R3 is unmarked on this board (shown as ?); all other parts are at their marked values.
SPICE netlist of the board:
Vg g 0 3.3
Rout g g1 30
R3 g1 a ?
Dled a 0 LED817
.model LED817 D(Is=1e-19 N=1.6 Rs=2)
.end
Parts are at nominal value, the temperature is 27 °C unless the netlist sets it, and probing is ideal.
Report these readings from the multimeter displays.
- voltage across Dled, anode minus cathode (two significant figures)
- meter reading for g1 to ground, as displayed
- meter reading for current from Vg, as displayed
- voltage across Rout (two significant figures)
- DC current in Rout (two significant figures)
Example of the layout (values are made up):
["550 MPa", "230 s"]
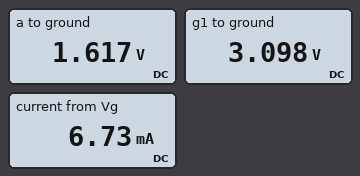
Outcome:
["1.6 V", "3.098 V", "6.73 mA", "200 mV", "6.7 mA"]
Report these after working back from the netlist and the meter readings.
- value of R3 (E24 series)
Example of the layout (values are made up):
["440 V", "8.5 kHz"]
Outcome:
["220 Ω"]
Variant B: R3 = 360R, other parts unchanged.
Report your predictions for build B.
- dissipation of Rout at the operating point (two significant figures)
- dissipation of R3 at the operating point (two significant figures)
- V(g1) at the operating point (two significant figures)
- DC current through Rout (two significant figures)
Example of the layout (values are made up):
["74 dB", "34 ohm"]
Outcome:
["570 µW", "6.9 mW", "3.2 V", "4.4 mA"]
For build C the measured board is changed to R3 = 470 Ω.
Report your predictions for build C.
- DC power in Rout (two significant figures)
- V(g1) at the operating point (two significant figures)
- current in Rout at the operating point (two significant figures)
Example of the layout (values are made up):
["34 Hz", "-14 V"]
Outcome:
["350 µW", "3.2 V", "3.4 mA"]
